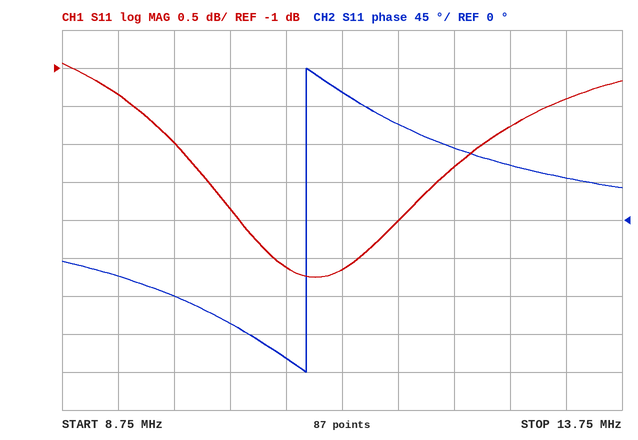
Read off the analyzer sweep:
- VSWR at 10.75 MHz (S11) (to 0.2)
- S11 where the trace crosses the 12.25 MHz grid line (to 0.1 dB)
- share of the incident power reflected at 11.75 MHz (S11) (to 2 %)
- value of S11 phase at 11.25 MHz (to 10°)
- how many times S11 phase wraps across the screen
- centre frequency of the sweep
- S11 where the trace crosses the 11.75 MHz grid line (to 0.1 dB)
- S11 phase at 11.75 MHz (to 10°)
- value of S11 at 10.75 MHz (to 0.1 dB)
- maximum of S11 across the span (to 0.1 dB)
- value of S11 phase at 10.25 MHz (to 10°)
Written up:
4.8
-2.3 dB
50 %
150°
1
11.25 MHz
-3.0 dB
110°
-3.6 dB
-0.9 dB
-120°
